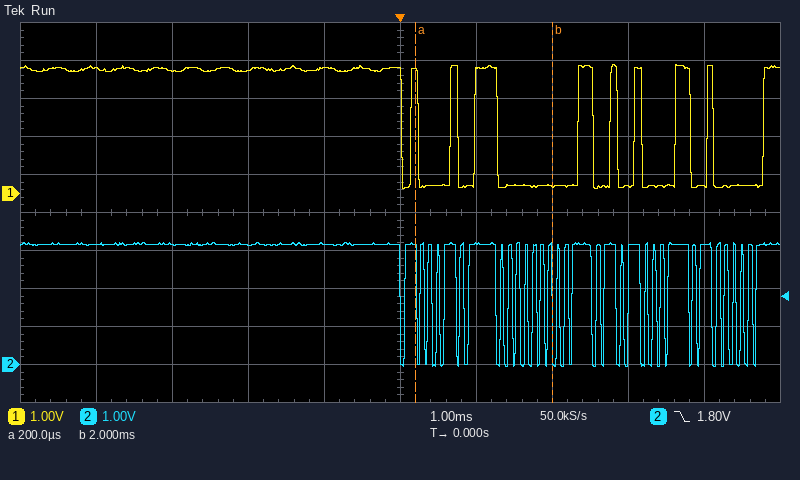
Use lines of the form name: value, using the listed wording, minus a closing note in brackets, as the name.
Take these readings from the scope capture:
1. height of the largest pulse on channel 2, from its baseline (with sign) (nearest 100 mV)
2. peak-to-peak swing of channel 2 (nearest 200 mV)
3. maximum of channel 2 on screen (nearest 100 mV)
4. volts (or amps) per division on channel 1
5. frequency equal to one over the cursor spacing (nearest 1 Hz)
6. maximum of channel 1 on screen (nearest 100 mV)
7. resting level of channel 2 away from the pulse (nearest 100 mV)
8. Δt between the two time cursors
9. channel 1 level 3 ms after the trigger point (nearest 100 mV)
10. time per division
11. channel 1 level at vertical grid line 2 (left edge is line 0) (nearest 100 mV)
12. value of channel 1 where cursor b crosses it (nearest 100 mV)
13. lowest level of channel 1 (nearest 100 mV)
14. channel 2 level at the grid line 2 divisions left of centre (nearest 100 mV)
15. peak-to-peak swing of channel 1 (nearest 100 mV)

height of the largest pulse on channel 2, from its baseline (with sign): -3.2 V
peak-to-peak swing of channel 2: 3.2 V
maximum of channel 2 on screen: 3.2 V
volts (or amps) per division on channel 1: 1 V
frequency equal to one over the cursor spacing: 556 Hz
maximum of channel 1 on screen: 3.4 V
resting level of channel 2 away from the pulse: 3.2 V
Δt between the two time cursors: 1.8 ms
channel 1 level 3 ms after the trigger point: 200 mV
time per division: 1 ms
channel 1 level at vertical grid line 2 (left edge is line 0): 3.2 V
value of channel 1 where cursor b crosses it: 200 mV
lowest level of channel 1: 100 mV
channel 2 level at the grid line 2 divisions left of centre: 3.1 V
peak-to-peak swing of channel 1: 3.3 V
